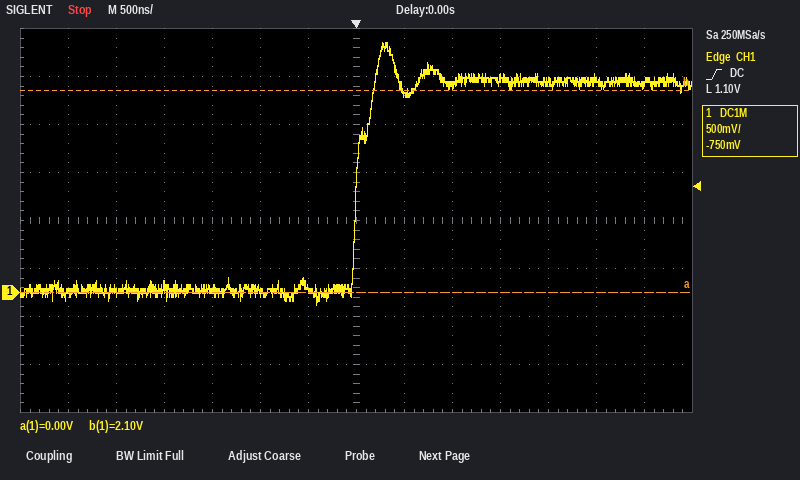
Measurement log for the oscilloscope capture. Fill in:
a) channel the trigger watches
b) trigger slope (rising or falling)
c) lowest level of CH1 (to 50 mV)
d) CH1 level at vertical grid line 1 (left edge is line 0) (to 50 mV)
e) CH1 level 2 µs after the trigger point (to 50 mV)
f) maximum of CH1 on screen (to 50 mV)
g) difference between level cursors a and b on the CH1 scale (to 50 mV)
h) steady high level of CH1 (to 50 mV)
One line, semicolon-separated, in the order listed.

CH1; rising; -100 mV; 0 mV; 2.20 V; 2.60 V; 2.10 V; 2.20 V
